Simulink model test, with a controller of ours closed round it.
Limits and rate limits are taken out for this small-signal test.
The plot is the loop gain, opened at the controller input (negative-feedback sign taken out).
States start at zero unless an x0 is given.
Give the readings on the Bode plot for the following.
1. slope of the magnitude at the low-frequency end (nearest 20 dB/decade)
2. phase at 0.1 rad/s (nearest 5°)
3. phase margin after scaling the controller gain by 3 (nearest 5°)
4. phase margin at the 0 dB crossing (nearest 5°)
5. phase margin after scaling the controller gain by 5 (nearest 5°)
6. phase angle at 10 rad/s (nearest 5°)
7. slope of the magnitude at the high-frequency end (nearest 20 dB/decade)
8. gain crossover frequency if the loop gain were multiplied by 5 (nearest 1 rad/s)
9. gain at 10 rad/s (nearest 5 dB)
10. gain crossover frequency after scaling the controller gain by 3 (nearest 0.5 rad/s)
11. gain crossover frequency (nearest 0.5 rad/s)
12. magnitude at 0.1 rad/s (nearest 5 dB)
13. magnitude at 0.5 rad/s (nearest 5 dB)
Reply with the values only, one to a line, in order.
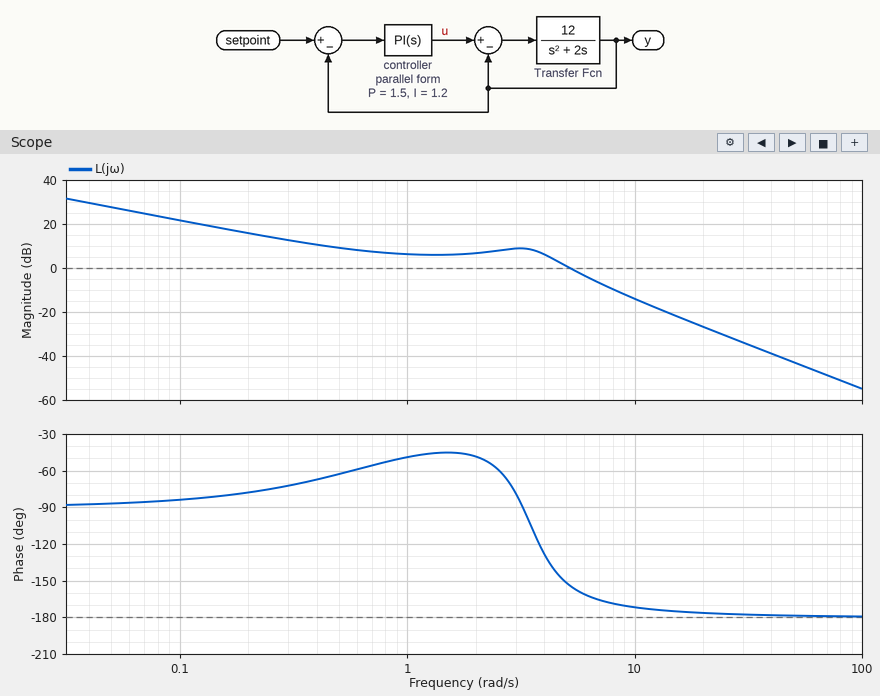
-20 dB/decade
-85°
10°
25°
10°
-170°
-40 dB/decade
10 rad/s
-15 dB
8.0 rad/s
5.0 rad/s
20 dB
10 dB
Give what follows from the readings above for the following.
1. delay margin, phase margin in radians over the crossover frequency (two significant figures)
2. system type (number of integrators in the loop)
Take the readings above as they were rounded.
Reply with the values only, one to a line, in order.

0.087 s
1
